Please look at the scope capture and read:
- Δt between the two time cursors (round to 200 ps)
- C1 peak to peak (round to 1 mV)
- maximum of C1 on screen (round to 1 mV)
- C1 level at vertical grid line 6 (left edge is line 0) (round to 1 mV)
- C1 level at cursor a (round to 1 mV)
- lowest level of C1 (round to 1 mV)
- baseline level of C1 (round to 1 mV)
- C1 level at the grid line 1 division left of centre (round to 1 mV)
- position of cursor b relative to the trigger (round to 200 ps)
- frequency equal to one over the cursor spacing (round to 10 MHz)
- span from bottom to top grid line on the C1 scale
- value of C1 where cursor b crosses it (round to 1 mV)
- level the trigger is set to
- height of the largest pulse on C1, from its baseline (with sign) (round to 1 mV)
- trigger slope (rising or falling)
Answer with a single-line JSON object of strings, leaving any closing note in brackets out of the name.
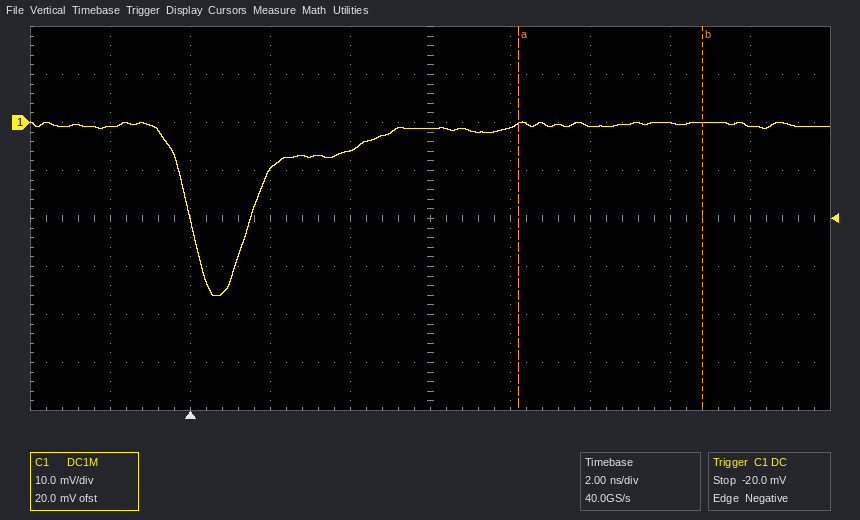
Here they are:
{"Δt between the two time cursors": "4.6 ns", "C1 peak to peak": "36 mV", "maximum of C1 on screen": "0 mV", "C1 level at vertical grid line 6 (left edge is line 0)": "-1 mV", "C1 level at cursor a": "0 mV", "lowest level of C1": "-36 mV", "baseline level of C1": "-1 mV", "C1 level at the grid line 1 division left of centre": "-6 mV", "position of cursor b relative to the trigger": "+12.8 ns", "frequency equal to one over the cursor spacing": "220 MHz", "span from bottom to top grid line on the C1 scale": "80 mV", "value of C1 where cursor b crosses it": "0 mV", "level the trigger is set to": "-20.0 mV", "height of the largest pulse on C1, from its baseline (with sign)": "-35 mV", "trigger slope": "falling"}
